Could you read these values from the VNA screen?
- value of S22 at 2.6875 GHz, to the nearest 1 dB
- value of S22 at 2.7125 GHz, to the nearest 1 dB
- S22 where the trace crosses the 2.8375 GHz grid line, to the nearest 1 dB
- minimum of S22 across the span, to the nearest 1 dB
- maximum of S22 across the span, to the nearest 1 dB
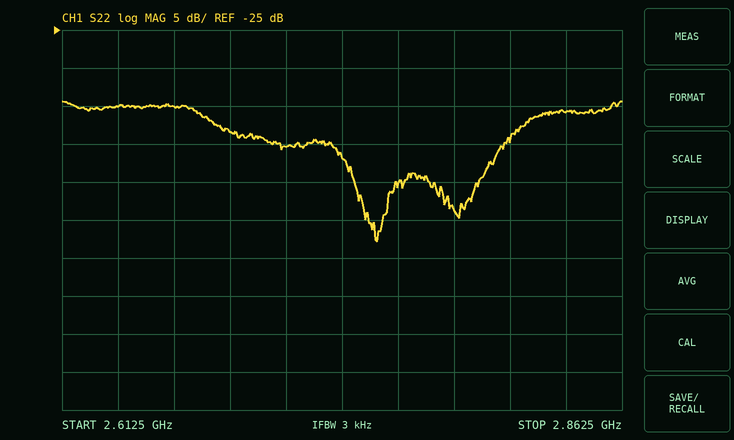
-38 dB
-40 dB
-36 dB
-53 dB
-34 dB
